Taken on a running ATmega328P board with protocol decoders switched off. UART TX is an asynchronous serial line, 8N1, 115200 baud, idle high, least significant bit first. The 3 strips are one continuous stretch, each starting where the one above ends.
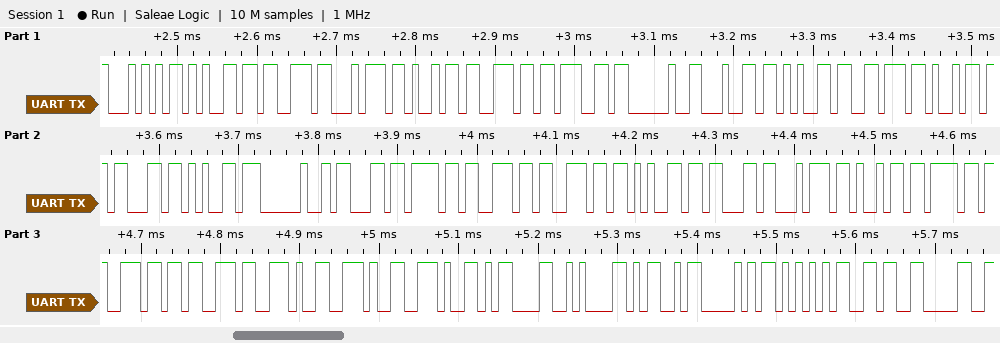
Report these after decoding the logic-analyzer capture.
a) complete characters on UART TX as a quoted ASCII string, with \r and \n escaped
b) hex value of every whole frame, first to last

"Testing device connections...\r\nMPU60"
54 65 73 74 69 6E 67 20 64 65 76 69 63 65 20 63 6F 6E 6E 65 63 74 69 6F 6E 73 2E 2E 2E 0D 0A 4D 50 55 36 30
